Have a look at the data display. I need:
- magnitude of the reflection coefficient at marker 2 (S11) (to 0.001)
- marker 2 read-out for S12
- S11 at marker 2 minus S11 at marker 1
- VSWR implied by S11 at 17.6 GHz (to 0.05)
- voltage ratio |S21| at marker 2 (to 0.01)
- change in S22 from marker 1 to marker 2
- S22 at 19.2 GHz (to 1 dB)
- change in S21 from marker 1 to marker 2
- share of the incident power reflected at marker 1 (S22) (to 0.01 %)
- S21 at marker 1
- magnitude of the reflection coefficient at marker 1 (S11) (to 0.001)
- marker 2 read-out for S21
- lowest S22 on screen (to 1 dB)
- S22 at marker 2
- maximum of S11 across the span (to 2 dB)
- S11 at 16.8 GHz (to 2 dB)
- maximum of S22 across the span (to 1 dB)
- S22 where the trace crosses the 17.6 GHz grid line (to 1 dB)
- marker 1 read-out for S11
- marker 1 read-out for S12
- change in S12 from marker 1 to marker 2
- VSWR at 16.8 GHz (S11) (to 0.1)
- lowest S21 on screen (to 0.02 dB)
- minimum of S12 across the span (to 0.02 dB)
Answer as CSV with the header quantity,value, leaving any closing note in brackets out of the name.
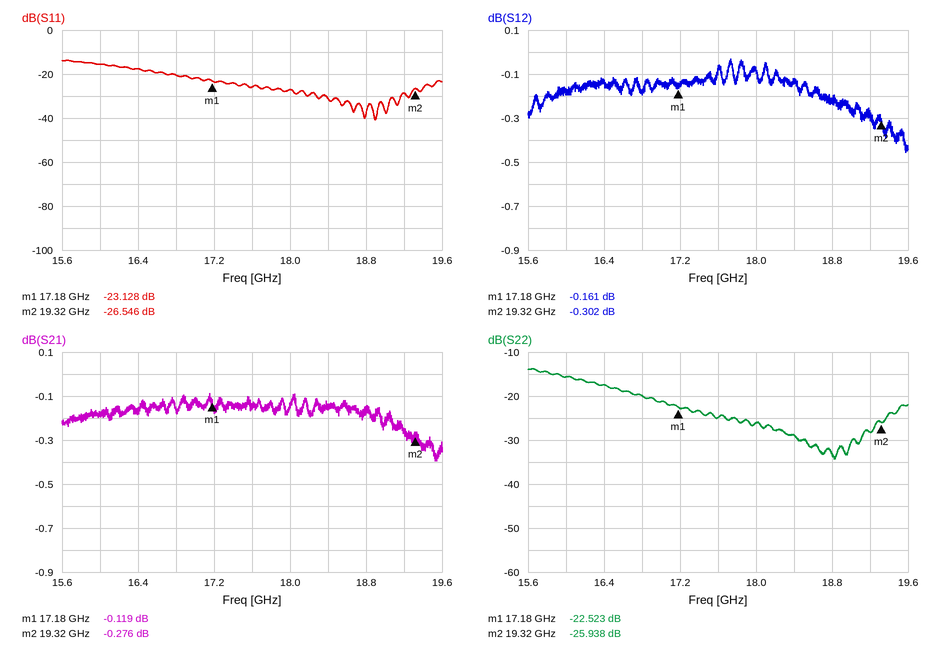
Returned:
quantity,value
magnitude of the reflection coefficient at marker 2 (S11),0.047
marker 2 read-out for S12,-0.302 dB
S11 at marker 2 minus S11 at marker 1,-3.418 dB
VSWR implied by S11 at 17.6 GHz,1.10
voltage ratio |S21| at marker 2,0.97
change in S22 from marker 1 to marker 2,-3.415 dB
S22 at 19.2 GHz,-28 dB
change in S21 from marker 1 to marker 2,-0.157 dB
share of the incident power reflected at marker 1 (S22),0.56 %
S21 at marker 1,-0.119 dB
magnitude of the reflection coefficient at marker 1 (S11),0.070
marker 2 read-out for S21,-0.276 dB
lowest S22 on screen,-34 dB
S22 at marker 2,-25.938 dB
maximum of S11 across the span,-14 dB
S11 at 16.8 GHz,-20 dB
maximum of S22 across the span,-14 dB
S22 where the trace crosses the 17.6 GHz grid line,-25 dB
marker 1 read-out for S11,-23.128 dB
marker 1 read-out for S12,-0.161 dB
change in S12 from marker 1 to marker 2,-0.141 dB
VSWR at 16.8 GHz (S11),1.2
lowest S21 on screen,-0.40 dB
minimum of S12 across the span,-0.46 dB
